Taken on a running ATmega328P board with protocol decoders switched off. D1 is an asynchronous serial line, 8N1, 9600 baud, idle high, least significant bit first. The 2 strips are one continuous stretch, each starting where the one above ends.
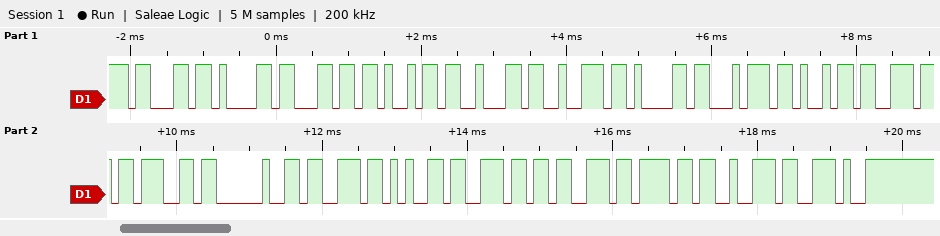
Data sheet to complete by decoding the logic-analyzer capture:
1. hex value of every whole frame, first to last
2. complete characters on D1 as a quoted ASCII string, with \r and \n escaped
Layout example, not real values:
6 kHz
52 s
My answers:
63 61 6C 69 62 72 61 74 69 6E 67 20 73 65 6E 73 6F 72 2E
"calibrating sensor."
